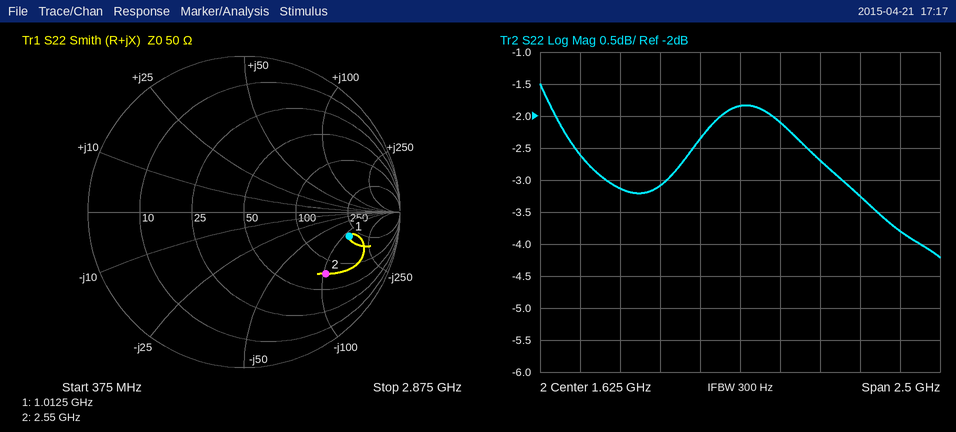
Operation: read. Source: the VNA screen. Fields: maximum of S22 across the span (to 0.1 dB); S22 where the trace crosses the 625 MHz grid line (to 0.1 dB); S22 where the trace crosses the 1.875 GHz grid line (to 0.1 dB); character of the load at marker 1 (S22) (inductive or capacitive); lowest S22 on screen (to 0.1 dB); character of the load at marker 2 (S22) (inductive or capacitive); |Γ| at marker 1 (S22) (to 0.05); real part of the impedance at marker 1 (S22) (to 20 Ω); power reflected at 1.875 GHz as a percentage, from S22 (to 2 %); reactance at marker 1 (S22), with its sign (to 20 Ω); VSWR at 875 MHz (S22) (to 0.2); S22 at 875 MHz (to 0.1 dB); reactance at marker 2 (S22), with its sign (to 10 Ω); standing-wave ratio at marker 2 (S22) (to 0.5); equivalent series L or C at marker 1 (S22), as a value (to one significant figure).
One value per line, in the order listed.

-1.5 dB
-2.6 dB
-2.1 dB
capacitive
-4.2 dB
capacitive
0.70
200 Ω
62 %
-120 Ω
5.6
-3.1 dB
-100 Ω
5.0
1 pF
